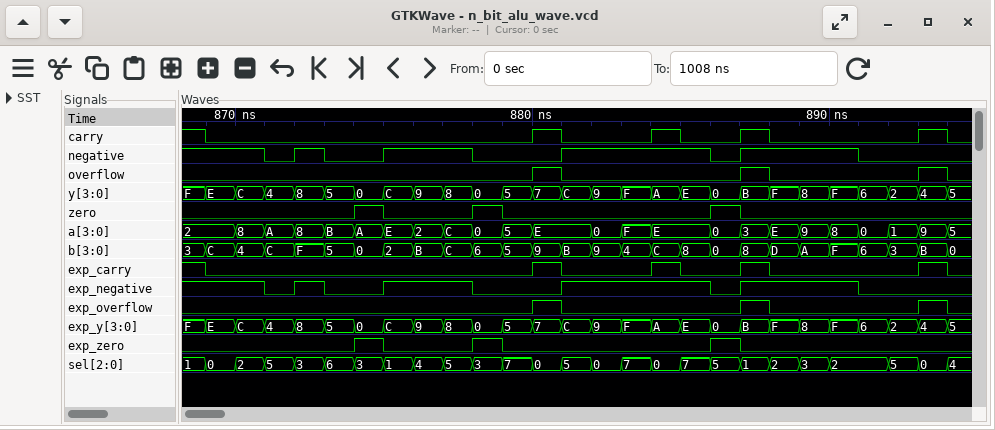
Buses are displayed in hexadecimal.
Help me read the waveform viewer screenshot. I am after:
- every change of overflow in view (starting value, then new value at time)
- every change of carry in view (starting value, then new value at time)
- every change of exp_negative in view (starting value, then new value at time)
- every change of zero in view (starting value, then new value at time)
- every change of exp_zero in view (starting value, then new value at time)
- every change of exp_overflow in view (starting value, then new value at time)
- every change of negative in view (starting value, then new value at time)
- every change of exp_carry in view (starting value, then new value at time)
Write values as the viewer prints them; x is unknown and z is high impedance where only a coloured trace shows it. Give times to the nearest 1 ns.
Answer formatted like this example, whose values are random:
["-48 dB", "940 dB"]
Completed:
["0, 1 at 880 ns, 0 at 881 ns, 1 at 887 ns, 0 at 888 ns, 1 at 893 ns, 0 at 894 ns", "1, 0 at 869 ns, 1 at 880 ns, 0 at 881 ns, 1 at 884 ns, 0 at 885 ns, 1 at 887 ns, 0 at 888 ns, 1 at 893 ns, 0 at 894 ns", "1, 0 at 871 ns, 1 at 872 ns, 0 at 873 ns, 1 at 875 ns, 0 at 878 ns, 1 at 881 ns, 0 at 886 ns, 1 at 887 ns, 0 at 891 ns", "0, 1 at 874 ns, 0 at 875 ns, 1 at 878 ns, 0 at 879 ns, 1 at 886 ns, 0 at 887 ns", "0, 1 at 874 ns, 0 at 875 ns, 1 at 878 ns, 0 at 879 ns, 1 at 886 ns, 0 at 887 ns", "0, 1 at 880 ns, 0 at 881 ns, 1 at 887 ns, 0 at 888 ns, 1 at 893 ns, 0 at 894 ns", "1, 0 at 871 ns, 1 at 872 ns, 0 at 873 ns, 1 at 875 ns, 0 at 878 ns, 1 at 881 ns, 0 at 886 ns, 1 at 887 ns, 0 at 891 ns", "1, 0 at 869 ns, 1 at 880 ns, 0 at 881 ns, 1 at 884 ns, 0 at 885 ns, 1 at 887 ns, 0 at 888 ns, 1 at 893 ns, 0 at 894 ns"]
